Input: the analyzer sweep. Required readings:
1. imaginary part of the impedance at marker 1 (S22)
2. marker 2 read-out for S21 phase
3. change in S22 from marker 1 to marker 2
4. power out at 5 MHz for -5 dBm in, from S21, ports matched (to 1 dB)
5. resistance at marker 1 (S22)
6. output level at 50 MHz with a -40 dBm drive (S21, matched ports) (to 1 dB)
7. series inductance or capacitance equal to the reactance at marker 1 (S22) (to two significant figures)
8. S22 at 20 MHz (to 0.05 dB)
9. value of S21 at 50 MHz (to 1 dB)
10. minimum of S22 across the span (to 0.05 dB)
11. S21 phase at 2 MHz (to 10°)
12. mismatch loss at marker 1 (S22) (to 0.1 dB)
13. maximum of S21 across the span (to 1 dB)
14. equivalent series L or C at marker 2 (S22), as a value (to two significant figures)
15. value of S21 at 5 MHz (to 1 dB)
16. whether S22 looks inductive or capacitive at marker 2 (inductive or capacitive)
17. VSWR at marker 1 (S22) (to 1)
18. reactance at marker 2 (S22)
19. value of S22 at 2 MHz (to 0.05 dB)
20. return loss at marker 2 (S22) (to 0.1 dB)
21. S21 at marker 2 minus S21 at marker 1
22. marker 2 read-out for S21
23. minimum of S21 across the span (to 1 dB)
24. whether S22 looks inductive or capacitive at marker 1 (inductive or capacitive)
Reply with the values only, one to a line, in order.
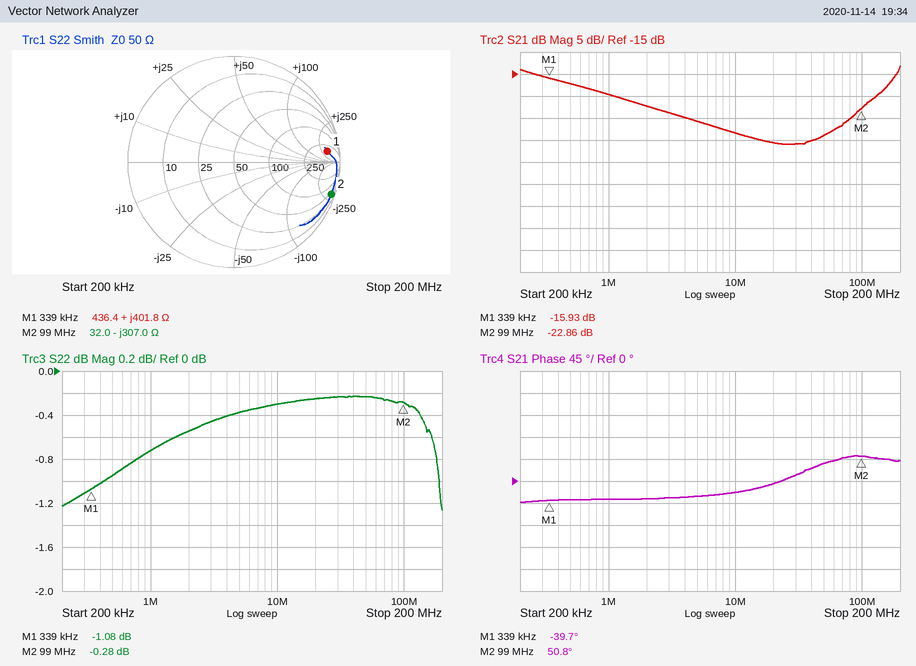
+401.8 Ω
50.8°
0.80 dB
-31 dBm
436.4 Ω
-69 dBm
190 µH
-0.25 dB
-29 dB
-1.25 dB
-40°
6.6 dB
-13 dB
5.2 pF
-26 dB
capacitive
16
-307.0 Ω
-0.55 dB
0.3 dB
-6.93 dB
-22.86 dB
-31 dB
inductive
